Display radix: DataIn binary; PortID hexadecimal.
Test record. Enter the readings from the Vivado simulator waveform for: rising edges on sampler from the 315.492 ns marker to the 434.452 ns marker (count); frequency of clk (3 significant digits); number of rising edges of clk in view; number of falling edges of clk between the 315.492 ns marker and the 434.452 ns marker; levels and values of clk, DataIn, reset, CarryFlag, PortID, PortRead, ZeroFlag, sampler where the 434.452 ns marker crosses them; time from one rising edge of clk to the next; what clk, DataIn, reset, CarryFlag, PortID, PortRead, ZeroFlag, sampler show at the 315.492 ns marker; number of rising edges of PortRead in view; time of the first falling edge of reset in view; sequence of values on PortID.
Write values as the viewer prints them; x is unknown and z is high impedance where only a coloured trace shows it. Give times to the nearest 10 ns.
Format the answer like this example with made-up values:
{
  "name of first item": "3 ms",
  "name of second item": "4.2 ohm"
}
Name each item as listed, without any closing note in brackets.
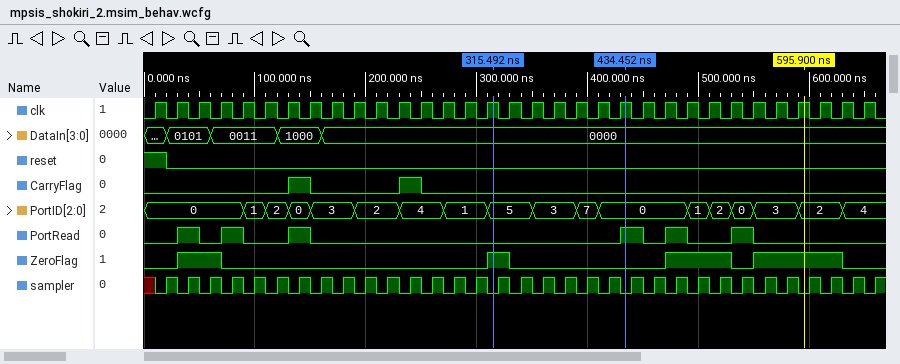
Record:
{
  "rising edges on sampler from the 315.492 ns marker to the 434.452 ns marker": "6",
  "frequency of clk": "50.0 MHz",
  "number of rising edges of clk in view": "33",
  "number of falling edges of clk between the 315.492 ns marker and the 434.452 ns marker": "6",
  "levels and values of clk, DataIn, reset, CarryFlag, PortID, PortRead, ZeroFlag, sampler where the 434.452 ns marker crosses them": "clk=1, DataIn=0000, reset=0, CarryFlag=0, PortID=0, PortRead=1, ZeroFlag=0, sampler=0",
  "time from one rising edge of clk to the next": "20 ns",
  "what clk, DataIn, reset, CarryFlag, PortID, PortRead, ZeroFlag, sampler show at the 315.492 ns marker": "clk=1, DataIn=0000, reset=0, CarryFlag=0, PortID=5, PortRead=0, ZeroFlag=1, sampler=0",
  "number of rising edges of PortRead in view": "6",
  "time of the first falling edge of reset in view": "20 ns",
  "sequence of values on PortID": "0, 1, 2, 0, 3, 2, 4, 1, 5, 3, 7, 0, 1, 2, 0, 3, 2, 4"
}
